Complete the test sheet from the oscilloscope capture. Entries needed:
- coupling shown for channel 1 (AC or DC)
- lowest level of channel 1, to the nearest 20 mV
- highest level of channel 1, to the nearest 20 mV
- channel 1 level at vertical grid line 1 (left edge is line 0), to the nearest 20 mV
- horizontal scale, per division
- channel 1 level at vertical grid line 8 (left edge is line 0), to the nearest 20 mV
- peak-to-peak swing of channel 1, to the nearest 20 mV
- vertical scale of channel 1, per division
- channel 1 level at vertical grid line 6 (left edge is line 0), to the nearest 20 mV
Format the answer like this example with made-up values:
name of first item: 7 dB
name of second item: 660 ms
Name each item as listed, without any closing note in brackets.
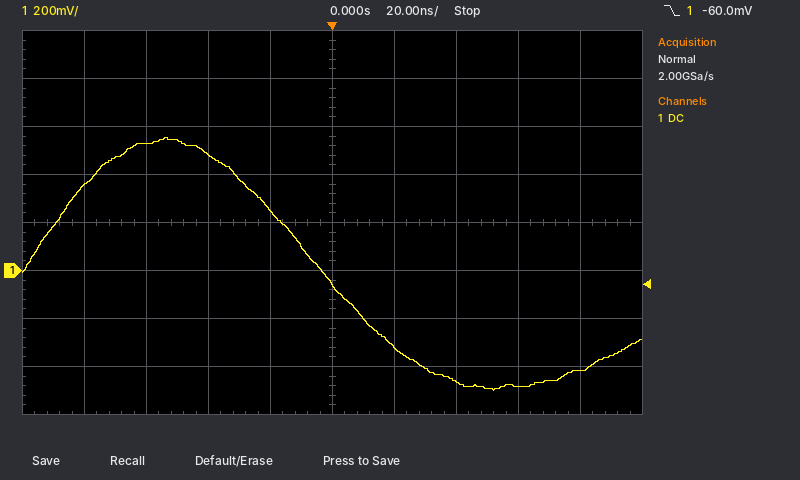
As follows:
coupling shown for channel 1: DC
lowest level of channel 1, to the nearest 20 mV: -500 mV
highest level of channel 1, to the nearest 20 mV: 560 mV
channel 1 level at vertical grid line 1 (left edge is line 0), to the nearest 20 mV: 360 mV
horizontal scale, per division: 20 ns
channel 1 level at vertical grid line 8 (left edge is line 0), to the nearest 20 mV: -480 mV
peak-to-peak swing of channel 1, to the nearest 20 mV: 1.06 V
vertical scale of channel 1, per division: 200 mV
channel 1 level at vertical grid line 6 (left edge is line 0), to the nearest 20 mV: -320 mV
